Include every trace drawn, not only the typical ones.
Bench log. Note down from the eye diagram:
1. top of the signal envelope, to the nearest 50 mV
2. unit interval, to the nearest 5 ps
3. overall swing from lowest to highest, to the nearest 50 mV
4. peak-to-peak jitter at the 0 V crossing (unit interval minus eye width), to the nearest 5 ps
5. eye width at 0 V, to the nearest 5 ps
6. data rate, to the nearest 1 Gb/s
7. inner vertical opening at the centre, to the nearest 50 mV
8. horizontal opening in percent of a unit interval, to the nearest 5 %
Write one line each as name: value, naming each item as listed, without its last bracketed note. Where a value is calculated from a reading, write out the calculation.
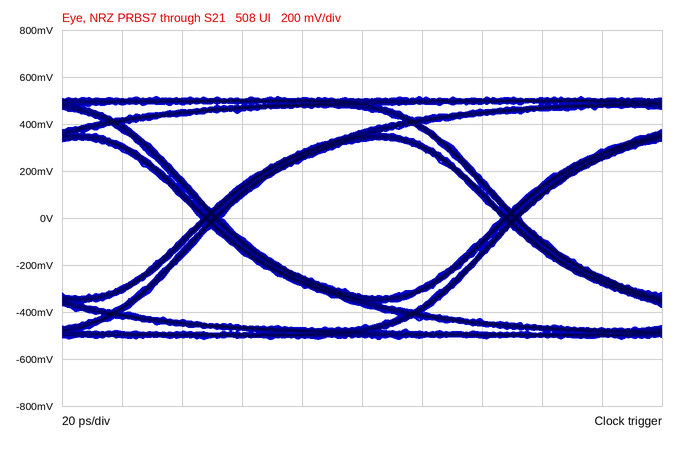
top of the signal envelope, to the nearest 50 mV: 500 mV
unit interval, to the nearest 5 ps: 100 ps
overall swing from lowest to highest, to the nearest 50 mV: 1.05 V
peak-to-peak jitter at the 0 V crossing (unit interval minus eye width), to the nearest 5 ps: 5 ps
eye width at 0 V, to the nearest 5 ps: 95 ps
data rate, to the nearest 1 Gb/s: 10 Gb/s
inner vertical opening at the centre, to the nearest 50 mV: 650 mV
horizontal opening in percent of a unit interval, to the nearest 5 %: 95 ps / 100 ps ≈ 95 %
